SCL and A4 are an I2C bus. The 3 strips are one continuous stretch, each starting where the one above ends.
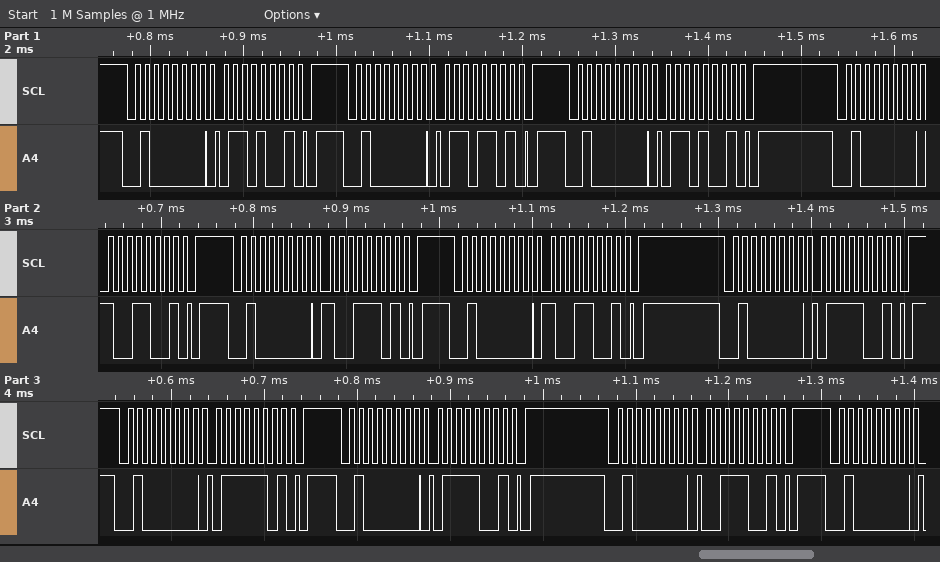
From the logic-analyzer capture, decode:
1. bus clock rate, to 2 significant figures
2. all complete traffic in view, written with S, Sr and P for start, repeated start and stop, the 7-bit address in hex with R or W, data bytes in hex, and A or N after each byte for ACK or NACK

100 kHz
S 20W A 69 A P S 20W A 6D A P S 20W A 69 A P S 20W A 99 A P S 20W A 9D A P S 20W A 99 A P S 20W A 79 A P S 20W A 7D A P S 20W A 79 A P S 20W A 39 A P S 20W A
